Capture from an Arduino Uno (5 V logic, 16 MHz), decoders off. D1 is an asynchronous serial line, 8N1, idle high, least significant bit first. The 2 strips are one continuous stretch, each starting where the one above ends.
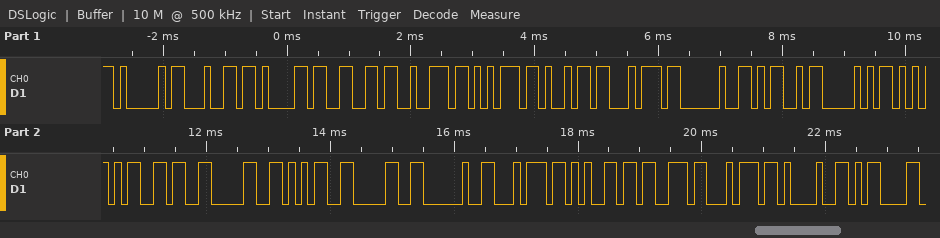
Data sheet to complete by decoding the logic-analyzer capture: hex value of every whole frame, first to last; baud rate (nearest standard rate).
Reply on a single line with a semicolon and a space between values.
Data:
41 64 61 66 72 75 69 74 20 4D 50 55 36 30 35 30 20 74 65 73 74 21 0D; 9600 baud
